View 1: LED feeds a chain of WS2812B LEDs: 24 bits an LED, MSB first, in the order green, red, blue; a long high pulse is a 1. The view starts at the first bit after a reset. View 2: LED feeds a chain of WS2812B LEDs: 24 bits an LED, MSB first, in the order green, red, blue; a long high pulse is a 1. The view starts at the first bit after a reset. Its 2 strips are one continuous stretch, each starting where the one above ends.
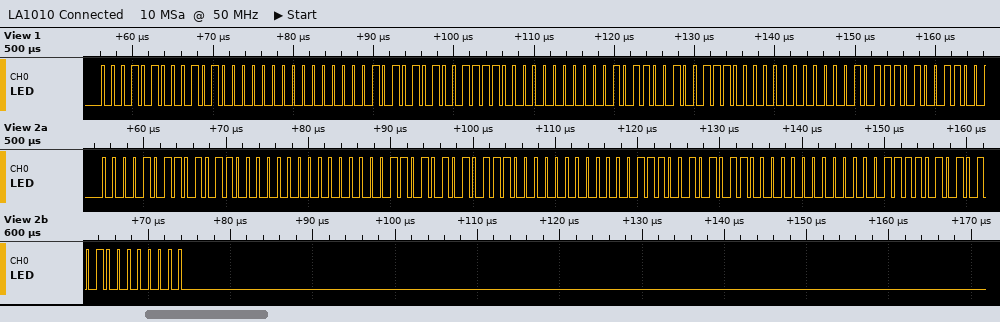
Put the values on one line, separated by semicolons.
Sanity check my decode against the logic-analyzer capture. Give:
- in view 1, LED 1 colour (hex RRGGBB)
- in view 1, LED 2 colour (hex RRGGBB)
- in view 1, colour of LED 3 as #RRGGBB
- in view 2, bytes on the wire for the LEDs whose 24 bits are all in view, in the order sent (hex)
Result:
#501400; #4F1500; #4E1600; 0B 58 00 0D 57 00 0E 56 00 0F 55 00
